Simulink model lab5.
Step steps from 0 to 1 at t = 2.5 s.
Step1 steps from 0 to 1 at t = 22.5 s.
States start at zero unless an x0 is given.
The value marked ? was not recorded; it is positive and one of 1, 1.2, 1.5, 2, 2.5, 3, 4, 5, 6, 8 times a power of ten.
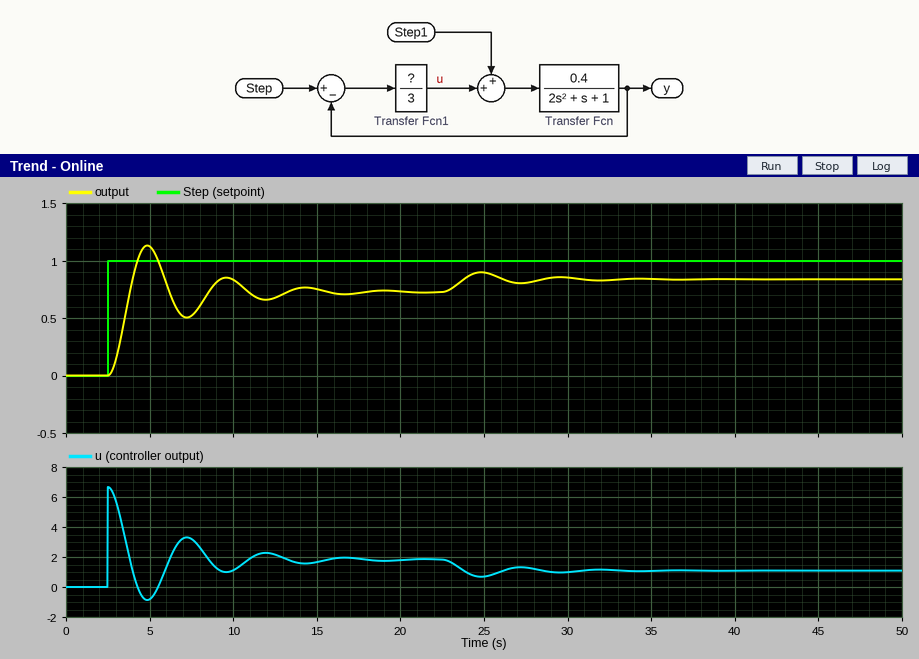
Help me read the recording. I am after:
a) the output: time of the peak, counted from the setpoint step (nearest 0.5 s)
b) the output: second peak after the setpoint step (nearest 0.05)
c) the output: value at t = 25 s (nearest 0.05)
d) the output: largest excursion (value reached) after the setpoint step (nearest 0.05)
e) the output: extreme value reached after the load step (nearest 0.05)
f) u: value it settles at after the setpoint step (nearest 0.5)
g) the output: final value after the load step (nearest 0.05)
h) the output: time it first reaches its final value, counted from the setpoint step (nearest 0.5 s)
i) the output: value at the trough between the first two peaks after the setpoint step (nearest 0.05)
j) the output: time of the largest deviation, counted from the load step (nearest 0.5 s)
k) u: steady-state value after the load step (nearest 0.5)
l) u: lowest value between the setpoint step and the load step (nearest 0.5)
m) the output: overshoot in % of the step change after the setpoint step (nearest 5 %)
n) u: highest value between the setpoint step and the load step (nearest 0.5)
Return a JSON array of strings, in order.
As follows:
["2.5 s", "0.85", "0.90", "1.15", "0.90", "2.0", "0.85", "1.5 s", "0.50", "2.5 s", "1.0", "-1.0", "55 %", "6.5"]
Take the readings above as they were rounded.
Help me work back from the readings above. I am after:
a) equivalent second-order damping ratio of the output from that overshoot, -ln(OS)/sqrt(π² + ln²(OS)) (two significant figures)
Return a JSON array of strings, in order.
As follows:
["0.19"]
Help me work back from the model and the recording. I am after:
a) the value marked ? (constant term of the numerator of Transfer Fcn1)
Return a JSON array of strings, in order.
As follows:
["20"]
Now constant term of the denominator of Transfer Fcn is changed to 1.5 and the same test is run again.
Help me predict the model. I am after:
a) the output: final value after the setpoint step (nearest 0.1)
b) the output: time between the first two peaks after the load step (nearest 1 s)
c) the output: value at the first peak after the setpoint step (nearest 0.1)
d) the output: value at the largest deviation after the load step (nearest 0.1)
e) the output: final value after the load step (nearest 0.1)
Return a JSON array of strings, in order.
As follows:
["0.6", "4 s", "1.0", "0.8", "0.7"]
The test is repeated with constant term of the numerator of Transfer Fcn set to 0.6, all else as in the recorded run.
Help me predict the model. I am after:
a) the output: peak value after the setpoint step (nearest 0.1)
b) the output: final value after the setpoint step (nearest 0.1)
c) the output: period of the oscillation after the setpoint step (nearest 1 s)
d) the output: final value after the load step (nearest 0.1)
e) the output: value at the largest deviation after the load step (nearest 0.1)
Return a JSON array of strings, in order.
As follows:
["1.3", "0.8", "4 s", "0.9", "1.0"]
